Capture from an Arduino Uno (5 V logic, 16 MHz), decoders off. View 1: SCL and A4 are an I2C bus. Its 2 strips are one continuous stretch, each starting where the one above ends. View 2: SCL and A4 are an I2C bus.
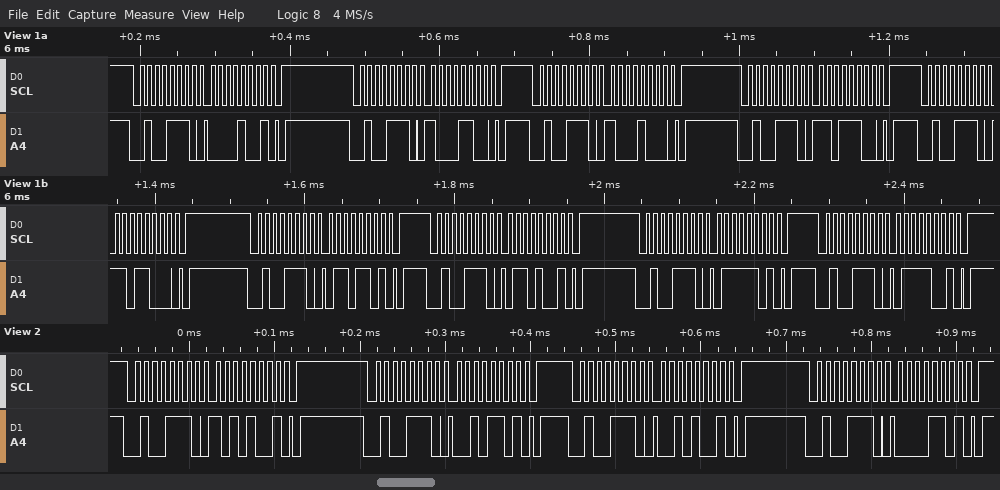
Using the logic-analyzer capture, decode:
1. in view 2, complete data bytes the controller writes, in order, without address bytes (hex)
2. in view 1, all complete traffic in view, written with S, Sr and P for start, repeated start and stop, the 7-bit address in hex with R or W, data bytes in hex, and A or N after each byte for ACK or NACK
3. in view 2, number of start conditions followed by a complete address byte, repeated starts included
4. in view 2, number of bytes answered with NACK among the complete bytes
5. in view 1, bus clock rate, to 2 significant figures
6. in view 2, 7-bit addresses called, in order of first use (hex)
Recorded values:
A9 2D 29 0D
S 27W A 09 A P S 27W A 8C A P S 27W A 88 A P S 27W A DC A P S 27W A D8 A P S 27W A 6D A P S 27W A 69 A P S 27W A 7D A P S 27W A 79 A P
4
0
100 kHz
0x27
